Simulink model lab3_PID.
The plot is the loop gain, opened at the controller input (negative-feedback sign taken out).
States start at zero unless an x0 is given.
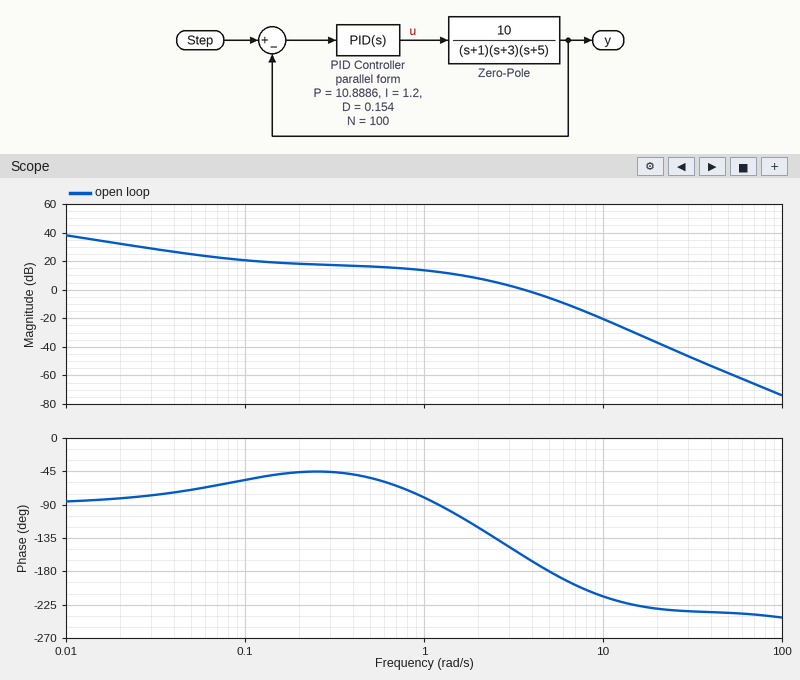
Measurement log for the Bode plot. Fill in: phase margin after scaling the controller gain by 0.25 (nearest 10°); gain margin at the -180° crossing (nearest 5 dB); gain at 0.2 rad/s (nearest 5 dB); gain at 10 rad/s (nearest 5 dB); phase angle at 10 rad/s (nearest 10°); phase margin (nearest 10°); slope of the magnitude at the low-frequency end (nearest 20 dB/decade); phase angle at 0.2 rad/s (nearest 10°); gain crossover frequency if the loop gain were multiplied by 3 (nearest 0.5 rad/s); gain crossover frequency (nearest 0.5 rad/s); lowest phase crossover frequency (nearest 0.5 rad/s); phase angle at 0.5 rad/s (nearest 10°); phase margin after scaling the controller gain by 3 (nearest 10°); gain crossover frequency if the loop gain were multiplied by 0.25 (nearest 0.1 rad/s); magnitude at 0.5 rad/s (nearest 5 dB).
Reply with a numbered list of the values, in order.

1. 90°
2. 5 dB
3. 20 dB
4. -20 dB
5. -210°
6. 20°
7. -20 dB/decade
8. -50°
9. 6.0 rad/s
10. 3.5 rad/s
11. 5.0 rad/s
12. -50°
13. -10°
14. 1.3 rad/s
15. 15 dB
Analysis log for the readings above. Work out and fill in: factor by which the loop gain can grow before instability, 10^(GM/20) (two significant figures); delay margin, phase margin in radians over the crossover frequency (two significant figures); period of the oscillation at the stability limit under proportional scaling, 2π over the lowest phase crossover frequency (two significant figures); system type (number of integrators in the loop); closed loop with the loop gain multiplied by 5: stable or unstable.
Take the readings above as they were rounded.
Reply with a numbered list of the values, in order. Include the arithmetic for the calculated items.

1. 10^(5 / 20) = 1.8
2. 20 × π / 180 / 3.5 = 0.100 s
3. 2π / 5 = 1.3 s
4. 1
5. unstable
